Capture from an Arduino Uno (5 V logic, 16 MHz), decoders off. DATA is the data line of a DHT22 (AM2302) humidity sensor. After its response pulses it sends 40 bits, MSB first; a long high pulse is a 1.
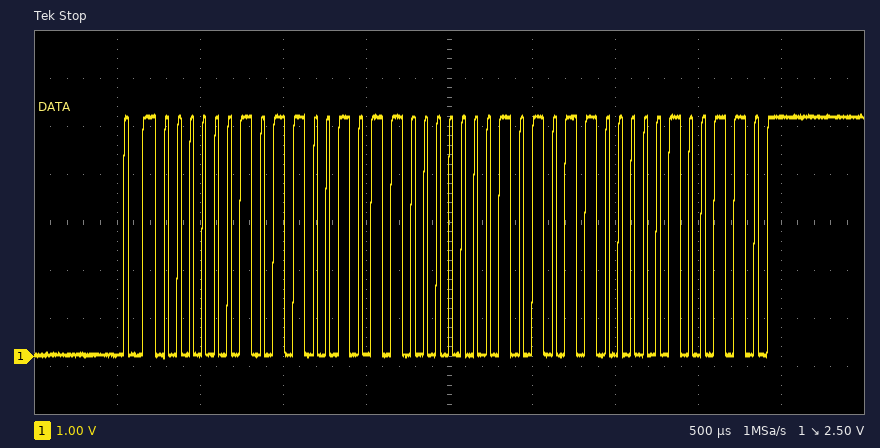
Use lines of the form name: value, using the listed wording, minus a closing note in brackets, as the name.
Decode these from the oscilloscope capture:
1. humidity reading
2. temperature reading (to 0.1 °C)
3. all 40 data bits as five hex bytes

humidity reading: 71.5 %
temperature reading: 34.4 °C
all 40 data bits as five hex bytes: 02 CB 01 58 26
